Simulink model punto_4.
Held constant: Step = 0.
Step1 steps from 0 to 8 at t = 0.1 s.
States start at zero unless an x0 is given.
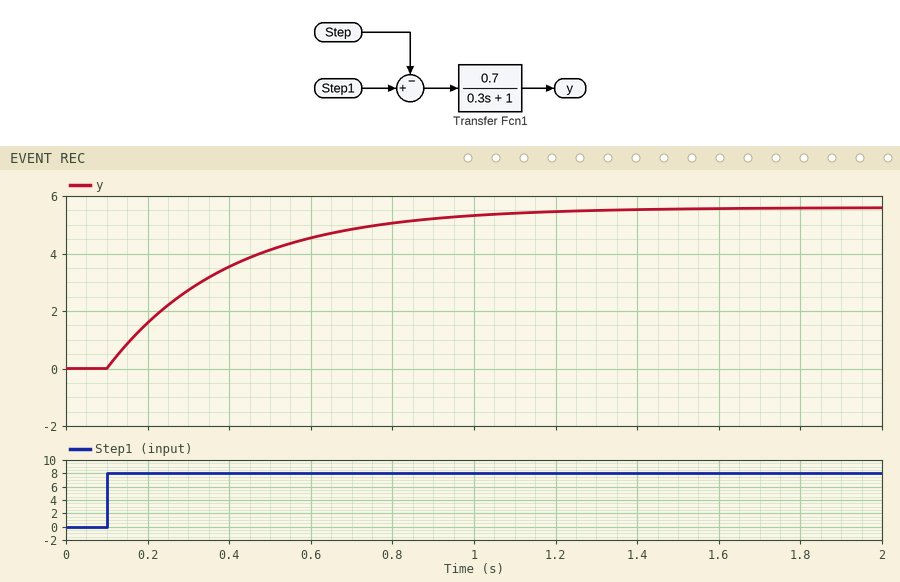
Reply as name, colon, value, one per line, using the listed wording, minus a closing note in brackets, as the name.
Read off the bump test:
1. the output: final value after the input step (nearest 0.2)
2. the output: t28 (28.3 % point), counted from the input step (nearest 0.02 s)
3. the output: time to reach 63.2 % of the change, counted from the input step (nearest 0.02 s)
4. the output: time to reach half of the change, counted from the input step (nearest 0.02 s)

the output: final value after the input step: 5.6
the output: t28 (28.3 % point), counted from the input step: 0.10 s
the output: time to reach 63.2 % of the change, counted from the input step: 0.30 s
the output: time to reach half of the change, counted from the input step: 0.20 s
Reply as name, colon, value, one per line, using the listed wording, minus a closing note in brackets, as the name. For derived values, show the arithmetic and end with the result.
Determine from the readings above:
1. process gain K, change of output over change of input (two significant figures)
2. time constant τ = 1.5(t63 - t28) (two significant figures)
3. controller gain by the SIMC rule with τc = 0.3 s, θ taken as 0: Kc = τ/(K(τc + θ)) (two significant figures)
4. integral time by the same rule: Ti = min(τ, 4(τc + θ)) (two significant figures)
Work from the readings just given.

process gain K, change of output over change of input: (5.6 - 0) / 8 = 0.70
time constant τ = 1.5(t63 - t28): 1.5 × (0.3 - 0.1) = 0.30 s
controller gain by the SIMC rule with τc = 0.3 s, θ taken as 0: Kc = τ/(K(τc + θ)): 0.3 / (0.7 × (0.3 + 0)) = 1.4
integral time by the same rule: Ti = min(τ, 4(τc + θ)): min(0.3, 4 × (0.3 + 0)) = 0.30 s
